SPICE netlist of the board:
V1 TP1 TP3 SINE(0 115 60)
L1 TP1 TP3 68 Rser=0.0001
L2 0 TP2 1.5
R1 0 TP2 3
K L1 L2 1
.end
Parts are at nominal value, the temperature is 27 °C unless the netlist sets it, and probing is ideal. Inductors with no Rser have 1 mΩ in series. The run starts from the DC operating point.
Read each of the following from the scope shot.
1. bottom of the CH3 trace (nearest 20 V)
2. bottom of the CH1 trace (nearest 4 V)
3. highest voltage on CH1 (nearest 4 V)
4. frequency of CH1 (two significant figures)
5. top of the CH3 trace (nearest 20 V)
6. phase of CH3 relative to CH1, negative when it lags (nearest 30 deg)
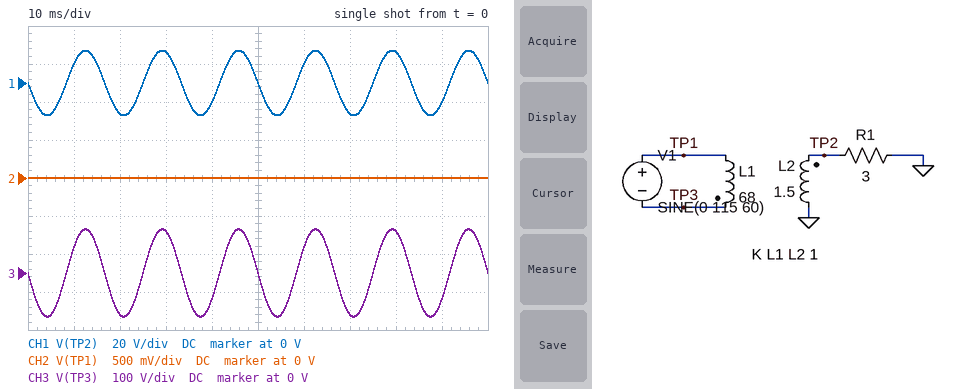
-120 V
-16 V
16 V
60 Hz
120 V
0 deg
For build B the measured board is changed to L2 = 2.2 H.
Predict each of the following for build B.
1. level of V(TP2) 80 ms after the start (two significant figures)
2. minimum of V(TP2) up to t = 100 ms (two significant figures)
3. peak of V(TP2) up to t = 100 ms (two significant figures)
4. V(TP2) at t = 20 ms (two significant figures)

20 V
-21 V
21 V
-20 V
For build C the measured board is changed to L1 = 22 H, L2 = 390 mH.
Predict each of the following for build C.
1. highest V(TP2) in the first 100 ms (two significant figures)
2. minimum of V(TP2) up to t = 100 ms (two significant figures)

15 V
-15 V
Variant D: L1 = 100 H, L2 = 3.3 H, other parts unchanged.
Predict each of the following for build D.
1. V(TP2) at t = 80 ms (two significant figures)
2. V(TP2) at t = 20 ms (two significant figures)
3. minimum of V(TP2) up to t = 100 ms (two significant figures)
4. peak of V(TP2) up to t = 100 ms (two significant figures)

20 V
-20 V
-21 V
21 V
